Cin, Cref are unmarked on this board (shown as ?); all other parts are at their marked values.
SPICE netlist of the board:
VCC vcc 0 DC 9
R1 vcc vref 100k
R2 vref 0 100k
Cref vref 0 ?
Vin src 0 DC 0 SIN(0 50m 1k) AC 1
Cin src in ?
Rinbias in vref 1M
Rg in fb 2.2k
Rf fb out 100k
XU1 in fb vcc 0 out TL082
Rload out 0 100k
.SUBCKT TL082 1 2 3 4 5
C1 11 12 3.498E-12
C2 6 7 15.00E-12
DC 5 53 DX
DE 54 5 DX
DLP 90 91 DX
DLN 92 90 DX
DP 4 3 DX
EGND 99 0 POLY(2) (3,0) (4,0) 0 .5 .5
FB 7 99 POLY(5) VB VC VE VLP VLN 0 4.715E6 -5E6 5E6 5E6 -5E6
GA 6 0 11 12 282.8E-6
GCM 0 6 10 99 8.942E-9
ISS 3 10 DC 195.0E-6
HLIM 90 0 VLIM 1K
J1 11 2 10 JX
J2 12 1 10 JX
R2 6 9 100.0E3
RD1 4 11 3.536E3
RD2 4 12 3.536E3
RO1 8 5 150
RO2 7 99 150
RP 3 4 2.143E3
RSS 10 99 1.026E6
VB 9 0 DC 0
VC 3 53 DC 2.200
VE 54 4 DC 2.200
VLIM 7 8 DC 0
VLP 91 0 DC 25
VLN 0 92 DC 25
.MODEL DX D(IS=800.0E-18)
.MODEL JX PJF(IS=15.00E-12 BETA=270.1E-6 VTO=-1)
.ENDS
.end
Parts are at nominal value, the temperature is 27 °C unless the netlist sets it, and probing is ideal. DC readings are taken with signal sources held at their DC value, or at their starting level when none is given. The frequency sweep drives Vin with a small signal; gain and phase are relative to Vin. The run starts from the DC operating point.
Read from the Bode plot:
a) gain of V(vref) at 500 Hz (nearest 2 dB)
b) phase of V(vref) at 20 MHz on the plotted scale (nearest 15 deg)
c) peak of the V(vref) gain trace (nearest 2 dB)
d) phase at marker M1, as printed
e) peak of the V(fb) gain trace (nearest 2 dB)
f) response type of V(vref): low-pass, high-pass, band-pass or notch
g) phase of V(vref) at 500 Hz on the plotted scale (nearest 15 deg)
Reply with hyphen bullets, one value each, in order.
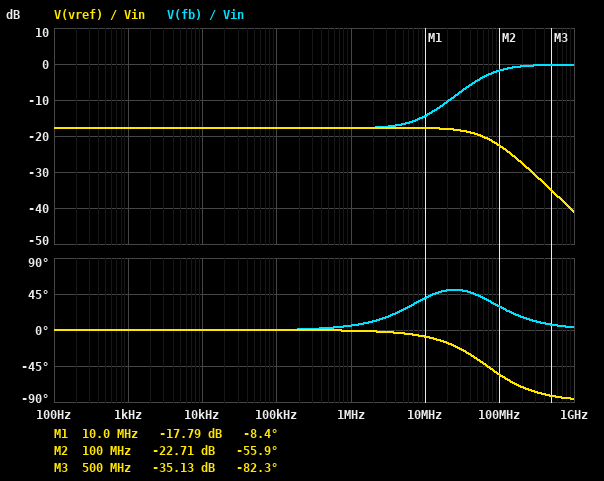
- -18 dB
- -15 deg
- -18 dB
- -8.4 deg
- 0 dB
- low-pass
- 0 deg
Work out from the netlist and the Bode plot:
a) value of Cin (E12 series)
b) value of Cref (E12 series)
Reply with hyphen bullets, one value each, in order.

- 2.7 µF
- 18 µF
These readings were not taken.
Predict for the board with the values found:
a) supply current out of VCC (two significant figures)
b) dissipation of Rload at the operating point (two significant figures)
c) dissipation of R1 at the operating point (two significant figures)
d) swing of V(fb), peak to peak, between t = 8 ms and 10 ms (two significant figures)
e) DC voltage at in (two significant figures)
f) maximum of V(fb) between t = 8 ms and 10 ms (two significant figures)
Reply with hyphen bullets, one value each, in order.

- 4.4 mA
- 200 µW
- 200 µW
- 13 mV
- 4.5 V
- 4.5 V
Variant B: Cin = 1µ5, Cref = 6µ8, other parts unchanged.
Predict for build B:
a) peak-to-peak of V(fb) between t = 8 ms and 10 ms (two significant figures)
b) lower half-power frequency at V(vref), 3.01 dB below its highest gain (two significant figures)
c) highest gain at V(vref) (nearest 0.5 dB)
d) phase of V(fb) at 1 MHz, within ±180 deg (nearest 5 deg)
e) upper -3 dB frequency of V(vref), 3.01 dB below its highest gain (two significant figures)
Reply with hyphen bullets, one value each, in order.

- 18 mV
- 380 mHz
- -15.0 dB
- 0 deg
- 130 MHz
